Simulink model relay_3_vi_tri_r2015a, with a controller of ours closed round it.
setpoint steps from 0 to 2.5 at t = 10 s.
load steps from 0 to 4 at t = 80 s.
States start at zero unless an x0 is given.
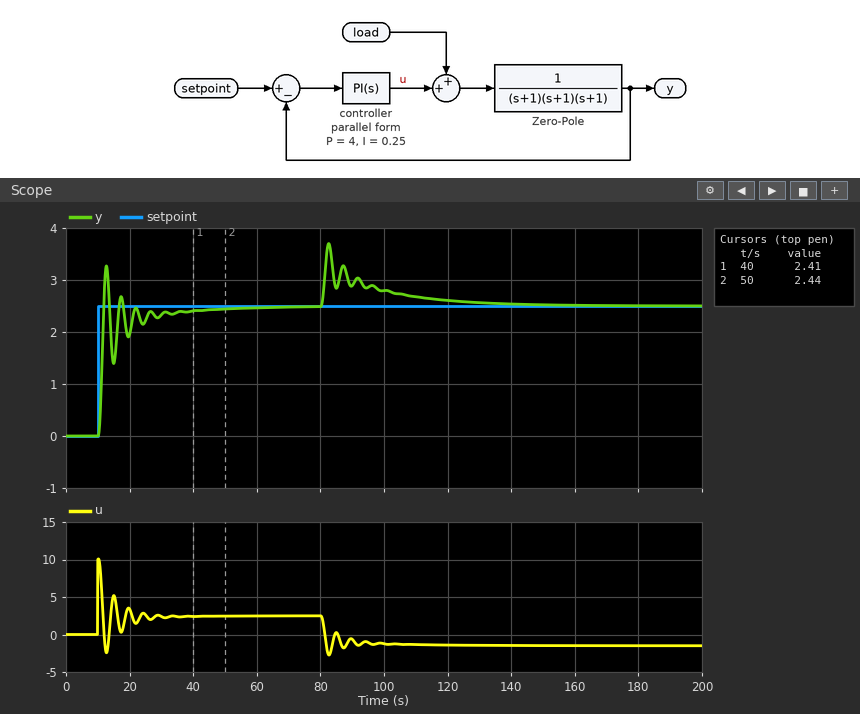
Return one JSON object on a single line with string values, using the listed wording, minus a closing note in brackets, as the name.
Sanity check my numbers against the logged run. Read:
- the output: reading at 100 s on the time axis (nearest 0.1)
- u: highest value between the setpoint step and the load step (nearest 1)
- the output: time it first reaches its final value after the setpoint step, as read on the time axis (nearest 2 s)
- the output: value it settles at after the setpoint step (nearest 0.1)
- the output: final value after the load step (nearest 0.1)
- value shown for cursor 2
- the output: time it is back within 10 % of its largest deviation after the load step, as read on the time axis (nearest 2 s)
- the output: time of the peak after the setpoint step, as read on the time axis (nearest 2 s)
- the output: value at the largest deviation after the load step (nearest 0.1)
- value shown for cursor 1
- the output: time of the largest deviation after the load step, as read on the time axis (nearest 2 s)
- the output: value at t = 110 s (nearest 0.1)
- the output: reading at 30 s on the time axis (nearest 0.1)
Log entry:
{"the output: reading at 100 s on the time axis": "2.8", "u: highest value between the setpoint step and the load step": "10", "the output: time it first reaches its final value after the setpoint step, as read on the time axis": "12 s", "the output: value it settles at after the setpoint step": "2.5", "the output: final value after the load step": "2.5", "value shown for cursor 2": "2.44", "the output: time it is back within 10 % of its largest deviation after the load step, as read on the time axis": "118 s", "the output: time of the peak after the setpoint step, as read on the time axis": "12 s", "the output: value at the largest deviation after the load step": "3.7", "value shown for cursor 1": "2.41", "the output: time of the largest deviation after the load step, as read on the time axis": "82 s", "the output: value at t = 110 s": "2.7", "the output: reading at 30 s on the time axis": "2.3"}
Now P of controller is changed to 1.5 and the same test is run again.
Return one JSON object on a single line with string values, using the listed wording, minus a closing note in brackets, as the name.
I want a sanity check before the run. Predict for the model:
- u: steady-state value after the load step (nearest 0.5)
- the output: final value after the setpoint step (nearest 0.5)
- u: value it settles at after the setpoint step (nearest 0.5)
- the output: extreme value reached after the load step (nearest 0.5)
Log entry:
{"u: steady-state value after the load step": "-1.5", "the output: final value after the setpoint step": "2.5", "u: value it settles at after the setpoint step": "2.5", "the output: extreme value reached after the load step": "4.5"}
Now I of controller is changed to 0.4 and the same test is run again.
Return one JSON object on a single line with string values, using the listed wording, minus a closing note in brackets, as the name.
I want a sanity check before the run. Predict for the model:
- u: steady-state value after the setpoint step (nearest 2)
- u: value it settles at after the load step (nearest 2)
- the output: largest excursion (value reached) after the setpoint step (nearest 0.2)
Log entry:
{"u: steady-state value after the setpoint step": "2", "u: value it settles at after the load step": "-2", "the output: largest excursion (value reached) after the setpoint step": "3.4"}
